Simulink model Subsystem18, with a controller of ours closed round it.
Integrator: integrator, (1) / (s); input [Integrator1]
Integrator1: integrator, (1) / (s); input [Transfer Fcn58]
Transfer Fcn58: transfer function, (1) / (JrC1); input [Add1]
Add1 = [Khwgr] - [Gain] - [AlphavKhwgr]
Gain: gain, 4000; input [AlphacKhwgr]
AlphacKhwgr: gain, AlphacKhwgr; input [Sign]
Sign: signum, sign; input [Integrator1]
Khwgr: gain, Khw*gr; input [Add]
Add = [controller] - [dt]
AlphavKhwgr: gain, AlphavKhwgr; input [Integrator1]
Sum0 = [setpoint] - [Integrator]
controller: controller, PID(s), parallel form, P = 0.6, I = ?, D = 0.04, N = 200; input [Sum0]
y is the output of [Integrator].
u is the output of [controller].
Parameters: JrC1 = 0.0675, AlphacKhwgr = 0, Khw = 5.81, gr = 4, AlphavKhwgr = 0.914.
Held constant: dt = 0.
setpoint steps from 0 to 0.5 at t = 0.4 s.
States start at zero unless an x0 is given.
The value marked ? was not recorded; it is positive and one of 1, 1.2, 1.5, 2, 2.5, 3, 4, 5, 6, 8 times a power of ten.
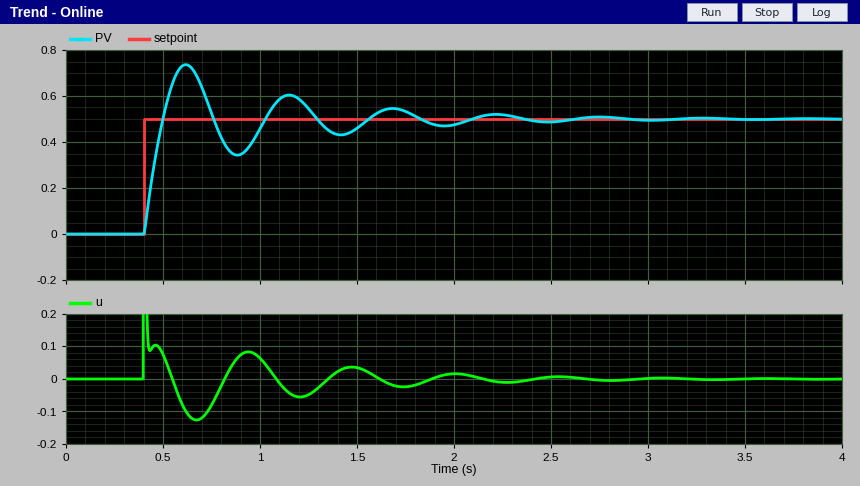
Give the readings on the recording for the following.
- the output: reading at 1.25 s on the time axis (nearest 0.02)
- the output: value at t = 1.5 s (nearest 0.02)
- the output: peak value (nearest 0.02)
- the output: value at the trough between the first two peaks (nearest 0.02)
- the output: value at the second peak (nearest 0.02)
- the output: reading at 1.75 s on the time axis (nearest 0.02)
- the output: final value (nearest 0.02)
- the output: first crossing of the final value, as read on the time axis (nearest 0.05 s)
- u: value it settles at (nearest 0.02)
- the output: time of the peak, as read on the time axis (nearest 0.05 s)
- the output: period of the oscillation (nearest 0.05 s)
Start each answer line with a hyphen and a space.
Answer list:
- 0.54
- 0.46
- 0.74
- 0.34
- 0.60
- 0.54
- 0.50
- 0.50 s
- 0.00
- 0.60 s
- 0.55 s
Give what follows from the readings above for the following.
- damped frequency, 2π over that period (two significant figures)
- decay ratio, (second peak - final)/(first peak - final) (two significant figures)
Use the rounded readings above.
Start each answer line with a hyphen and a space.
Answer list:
- 11 rad/s
- 0.42
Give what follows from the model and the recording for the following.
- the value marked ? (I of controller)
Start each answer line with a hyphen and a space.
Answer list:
- 10
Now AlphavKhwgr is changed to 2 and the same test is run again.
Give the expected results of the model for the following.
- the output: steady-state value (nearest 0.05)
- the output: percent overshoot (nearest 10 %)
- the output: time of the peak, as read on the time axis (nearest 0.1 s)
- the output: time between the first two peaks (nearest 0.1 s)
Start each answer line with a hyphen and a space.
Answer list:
- 0.50
- 50 %
- 0.7 s
- 0.7 s
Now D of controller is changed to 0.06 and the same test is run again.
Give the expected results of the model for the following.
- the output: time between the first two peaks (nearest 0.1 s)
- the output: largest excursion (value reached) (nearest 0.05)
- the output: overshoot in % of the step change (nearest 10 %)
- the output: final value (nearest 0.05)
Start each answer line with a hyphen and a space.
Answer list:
- 0.6 s
- 0.65
- 30 %
- 0.50
